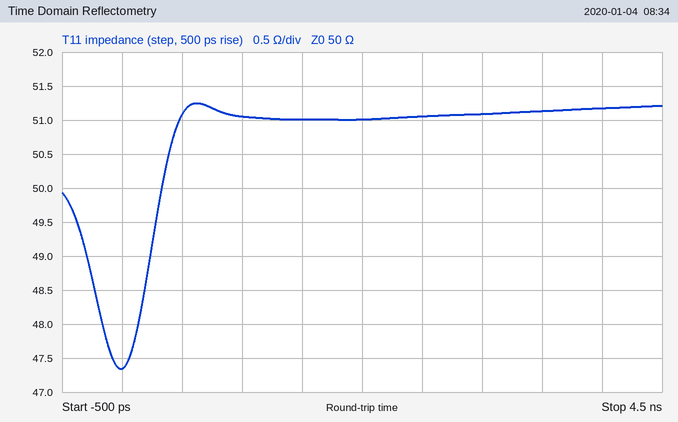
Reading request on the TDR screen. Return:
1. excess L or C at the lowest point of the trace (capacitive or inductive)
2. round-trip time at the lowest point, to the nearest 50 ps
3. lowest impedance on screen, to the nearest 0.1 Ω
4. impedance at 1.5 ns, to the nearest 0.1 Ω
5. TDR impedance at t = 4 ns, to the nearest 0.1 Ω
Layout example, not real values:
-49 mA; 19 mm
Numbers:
capacitive; 0 ps; 47.3 Ω; 51.0 Ω; 51.2 Ω
